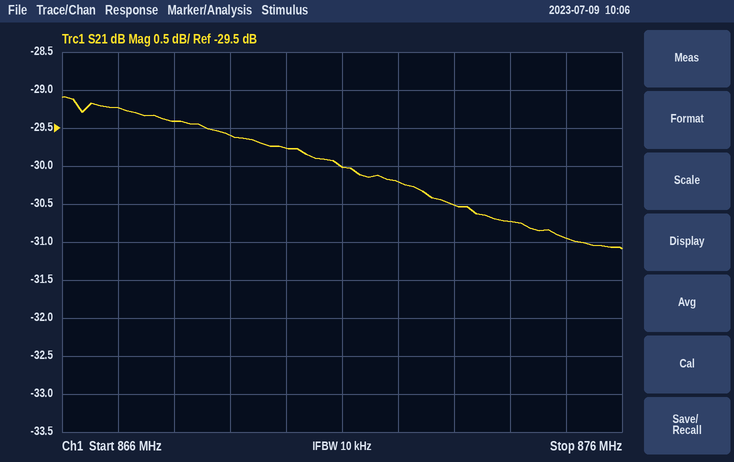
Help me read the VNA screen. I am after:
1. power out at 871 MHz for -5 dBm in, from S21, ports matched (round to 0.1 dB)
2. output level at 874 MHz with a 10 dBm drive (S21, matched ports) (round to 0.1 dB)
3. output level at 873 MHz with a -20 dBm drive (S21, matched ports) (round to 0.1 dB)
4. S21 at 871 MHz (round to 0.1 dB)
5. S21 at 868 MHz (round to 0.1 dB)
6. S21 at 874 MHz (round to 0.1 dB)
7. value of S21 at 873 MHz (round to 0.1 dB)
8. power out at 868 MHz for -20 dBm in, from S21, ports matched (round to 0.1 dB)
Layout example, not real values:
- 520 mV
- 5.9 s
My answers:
- -35.0 dBm
- -20.7 dBm
- -50.5 dBm
- -30.0 dB
- -29.4 dB
- -30.7 dB
- -30.5 dB
- -49.4 dBm
